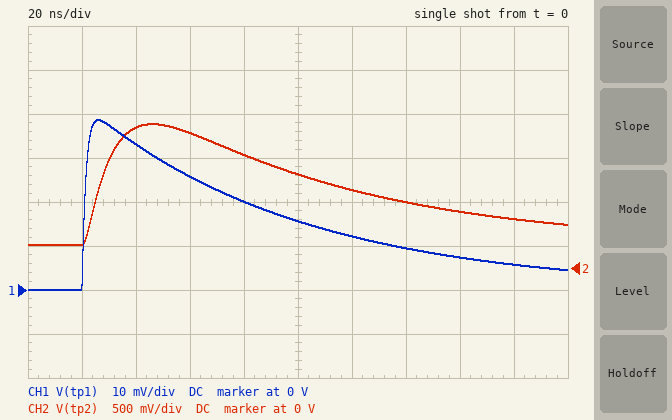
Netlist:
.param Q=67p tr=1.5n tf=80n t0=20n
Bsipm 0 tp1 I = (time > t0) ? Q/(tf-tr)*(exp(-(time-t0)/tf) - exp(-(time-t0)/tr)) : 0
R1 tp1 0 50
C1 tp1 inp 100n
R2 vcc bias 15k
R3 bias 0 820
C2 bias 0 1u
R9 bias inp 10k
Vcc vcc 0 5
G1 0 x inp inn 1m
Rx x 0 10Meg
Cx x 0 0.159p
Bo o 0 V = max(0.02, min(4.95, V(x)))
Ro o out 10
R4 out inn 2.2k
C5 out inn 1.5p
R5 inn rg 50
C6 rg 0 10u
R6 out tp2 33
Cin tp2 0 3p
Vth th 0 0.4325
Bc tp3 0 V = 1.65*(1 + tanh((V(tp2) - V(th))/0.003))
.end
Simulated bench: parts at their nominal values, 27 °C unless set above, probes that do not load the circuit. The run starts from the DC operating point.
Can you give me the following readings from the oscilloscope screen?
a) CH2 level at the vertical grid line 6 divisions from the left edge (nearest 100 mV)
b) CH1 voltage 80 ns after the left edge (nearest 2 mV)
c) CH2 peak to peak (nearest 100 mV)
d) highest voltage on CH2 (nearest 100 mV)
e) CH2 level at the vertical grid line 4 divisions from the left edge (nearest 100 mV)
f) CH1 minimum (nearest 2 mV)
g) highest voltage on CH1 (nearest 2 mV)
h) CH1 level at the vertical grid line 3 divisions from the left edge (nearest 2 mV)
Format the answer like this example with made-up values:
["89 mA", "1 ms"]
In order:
["900 mV", "20 mV", "1.4 V", "1.6 V", "1.3 V", "0 V", "38 mV", "26 mV"]
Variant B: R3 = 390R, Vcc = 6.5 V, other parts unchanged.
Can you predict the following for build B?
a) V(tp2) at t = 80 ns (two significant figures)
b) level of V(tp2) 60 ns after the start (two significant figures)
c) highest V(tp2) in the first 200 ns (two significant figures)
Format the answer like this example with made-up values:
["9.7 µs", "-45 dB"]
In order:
["1.2 V", "1.4 V", "1.5 V"]
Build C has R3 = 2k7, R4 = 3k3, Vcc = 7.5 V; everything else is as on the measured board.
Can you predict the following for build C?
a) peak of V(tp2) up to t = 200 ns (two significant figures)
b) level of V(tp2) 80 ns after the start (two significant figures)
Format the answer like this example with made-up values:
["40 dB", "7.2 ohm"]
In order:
["3.0 V", "2.7 V"]
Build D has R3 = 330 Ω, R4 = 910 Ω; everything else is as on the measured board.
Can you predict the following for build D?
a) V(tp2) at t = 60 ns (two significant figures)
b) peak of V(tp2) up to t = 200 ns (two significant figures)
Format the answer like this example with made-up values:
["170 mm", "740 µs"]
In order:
["630 mV", "780 mV"]
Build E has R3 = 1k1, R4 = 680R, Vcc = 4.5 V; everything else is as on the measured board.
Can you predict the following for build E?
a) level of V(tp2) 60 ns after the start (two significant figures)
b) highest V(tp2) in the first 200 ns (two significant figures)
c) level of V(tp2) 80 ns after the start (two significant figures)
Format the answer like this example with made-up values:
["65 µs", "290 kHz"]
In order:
["700 mV", "830 mV", "610 mV"]
